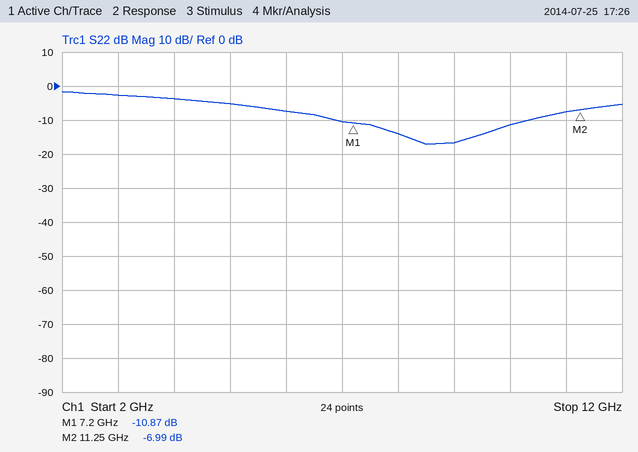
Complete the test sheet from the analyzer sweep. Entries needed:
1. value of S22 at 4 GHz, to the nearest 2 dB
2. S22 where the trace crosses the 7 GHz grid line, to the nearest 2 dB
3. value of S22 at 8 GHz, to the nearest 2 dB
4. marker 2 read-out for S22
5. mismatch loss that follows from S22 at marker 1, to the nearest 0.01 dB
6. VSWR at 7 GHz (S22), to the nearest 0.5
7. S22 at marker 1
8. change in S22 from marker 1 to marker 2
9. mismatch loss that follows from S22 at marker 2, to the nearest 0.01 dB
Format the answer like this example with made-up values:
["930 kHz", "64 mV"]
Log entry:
["-4 dB", "-10 dB", "-14 dB", "-6.99 dB", "0.37 dB", "2.0", "-10.87 dB", "3.88 dB", "0.97 dB"]
